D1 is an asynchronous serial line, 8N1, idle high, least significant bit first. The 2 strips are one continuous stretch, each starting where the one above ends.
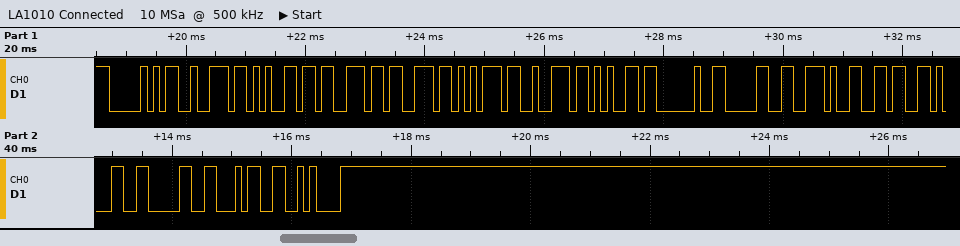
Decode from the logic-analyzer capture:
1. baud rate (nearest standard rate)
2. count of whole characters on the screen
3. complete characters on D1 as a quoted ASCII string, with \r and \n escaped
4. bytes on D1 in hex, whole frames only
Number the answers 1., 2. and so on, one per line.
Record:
1. 9600 baud
2. 16
3. "Pressure 0.6104\n"
4. 0x50 0x72 0x65 0x73 0x73 0x75 0x72 0x65 0x20 0x30 0x2E 0x36 0x31 0x30 0x34 0x0A
